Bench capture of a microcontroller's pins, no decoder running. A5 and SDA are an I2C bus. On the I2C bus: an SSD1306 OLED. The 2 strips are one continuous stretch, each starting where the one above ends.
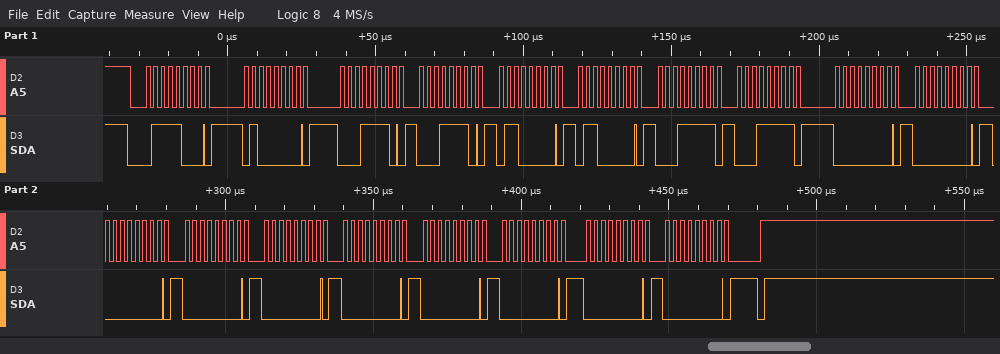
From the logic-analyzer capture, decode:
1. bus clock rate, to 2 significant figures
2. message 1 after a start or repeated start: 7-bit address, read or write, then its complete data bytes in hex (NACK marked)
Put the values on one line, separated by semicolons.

400 kHz; 0x3C write: 40 1E 1E 60 60 1F 1F 00 00 00 00 00 00 00 00 00 00
